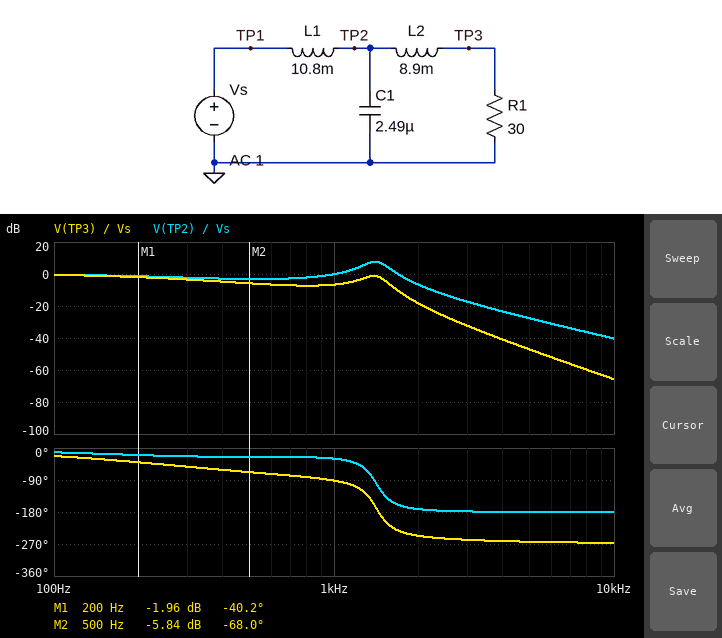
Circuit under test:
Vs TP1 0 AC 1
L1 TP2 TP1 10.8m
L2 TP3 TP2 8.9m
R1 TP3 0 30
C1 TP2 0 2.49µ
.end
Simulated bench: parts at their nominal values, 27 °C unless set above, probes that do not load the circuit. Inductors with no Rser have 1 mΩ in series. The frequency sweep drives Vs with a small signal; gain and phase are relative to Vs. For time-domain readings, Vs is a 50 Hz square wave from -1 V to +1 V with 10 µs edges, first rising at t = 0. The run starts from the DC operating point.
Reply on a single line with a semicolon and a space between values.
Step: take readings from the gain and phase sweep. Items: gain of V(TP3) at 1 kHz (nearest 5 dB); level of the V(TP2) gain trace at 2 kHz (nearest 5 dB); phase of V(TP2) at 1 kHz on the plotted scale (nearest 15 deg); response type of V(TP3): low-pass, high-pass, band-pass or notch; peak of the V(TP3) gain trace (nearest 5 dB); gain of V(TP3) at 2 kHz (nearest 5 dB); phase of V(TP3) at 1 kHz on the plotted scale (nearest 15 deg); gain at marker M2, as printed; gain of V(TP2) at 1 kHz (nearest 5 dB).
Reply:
-5 dB; -5 dB; -30 deg; low-pass; 0 dB; -20 dB; -90 deg; -5.84 dB; 0 dB
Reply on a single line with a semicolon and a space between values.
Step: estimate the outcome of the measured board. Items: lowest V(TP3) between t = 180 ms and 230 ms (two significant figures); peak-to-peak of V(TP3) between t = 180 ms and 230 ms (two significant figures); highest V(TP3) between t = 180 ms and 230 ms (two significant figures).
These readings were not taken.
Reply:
-1.0 V; 2.0 V; 1.0 V
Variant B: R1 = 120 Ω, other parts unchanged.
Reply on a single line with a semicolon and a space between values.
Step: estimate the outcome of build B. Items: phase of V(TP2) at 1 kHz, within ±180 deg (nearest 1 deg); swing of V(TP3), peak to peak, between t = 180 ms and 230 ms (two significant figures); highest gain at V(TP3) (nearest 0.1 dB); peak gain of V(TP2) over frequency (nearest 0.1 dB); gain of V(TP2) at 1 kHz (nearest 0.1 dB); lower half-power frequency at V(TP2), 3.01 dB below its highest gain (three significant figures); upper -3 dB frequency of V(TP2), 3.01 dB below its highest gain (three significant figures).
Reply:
-72 deg; 3.5 V; 5.4 dB; 6.3 dB; 6.2 dB; 715 Hz; 1.28 kHz
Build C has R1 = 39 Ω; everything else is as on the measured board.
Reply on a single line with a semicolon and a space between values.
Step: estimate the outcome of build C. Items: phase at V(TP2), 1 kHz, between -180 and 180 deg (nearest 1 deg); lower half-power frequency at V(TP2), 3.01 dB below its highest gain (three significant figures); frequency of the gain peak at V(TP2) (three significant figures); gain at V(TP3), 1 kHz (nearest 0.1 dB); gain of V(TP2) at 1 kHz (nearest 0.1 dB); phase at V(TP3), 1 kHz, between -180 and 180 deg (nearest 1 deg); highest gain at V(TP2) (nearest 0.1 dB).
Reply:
-37 deg; 1.17 kHz; 1.37 kHz; -4.4 dB; 0.5 dB; -92 deg; 6.2 dB
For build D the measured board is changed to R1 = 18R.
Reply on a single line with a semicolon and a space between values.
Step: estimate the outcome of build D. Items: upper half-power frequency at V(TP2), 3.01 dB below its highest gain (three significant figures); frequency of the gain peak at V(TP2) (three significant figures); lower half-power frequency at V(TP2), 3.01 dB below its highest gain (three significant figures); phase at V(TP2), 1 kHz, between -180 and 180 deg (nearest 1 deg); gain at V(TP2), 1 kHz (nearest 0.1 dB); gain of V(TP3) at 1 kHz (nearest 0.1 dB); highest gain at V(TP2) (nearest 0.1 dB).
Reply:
1.51 kHz; 1.43 kHz; 1.34 kHz; -19 deg; -0.8 dB; -11.1 dB; 11.7 dB
